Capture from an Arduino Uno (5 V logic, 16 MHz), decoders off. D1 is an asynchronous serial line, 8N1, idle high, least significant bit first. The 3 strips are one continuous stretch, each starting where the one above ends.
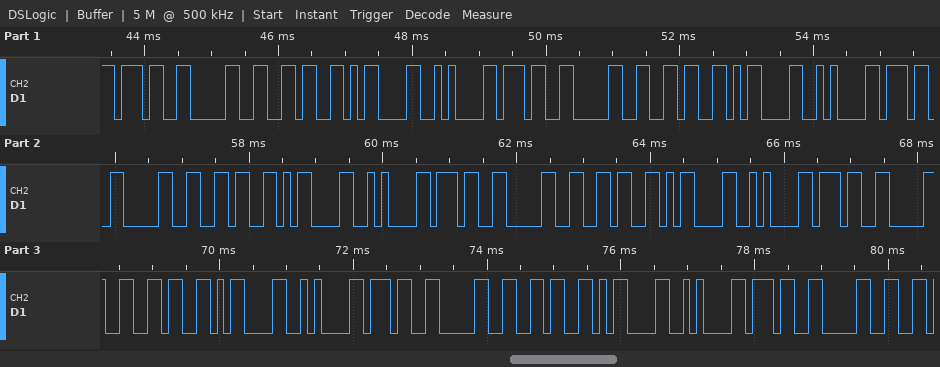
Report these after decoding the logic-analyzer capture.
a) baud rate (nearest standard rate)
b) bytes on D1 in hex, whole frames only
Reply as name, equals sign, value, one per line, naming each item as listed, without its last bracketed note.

baud rate = 9600 baud
bytes on D1 in hex, whole frames only = 0x37 0x30 0x36 0x0D 0x0A 0x37 0x30 0x36 0x0D 0x0A 0x37 0x30 0x36 0x0D 0x0A 0x37 0x30 0x36 0x0D 0x0A 0x37 0x30 0x36 0x0D 0x0A 0x37 0x30 0x36 0x0D 0x0A 0x37 0x30
